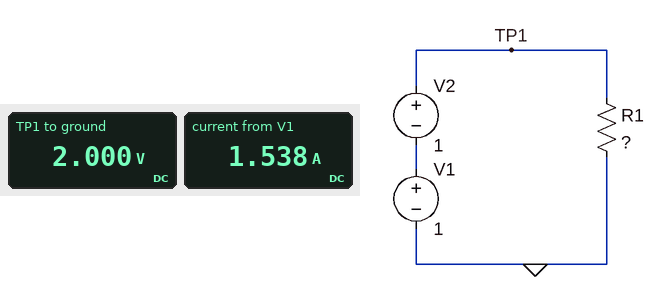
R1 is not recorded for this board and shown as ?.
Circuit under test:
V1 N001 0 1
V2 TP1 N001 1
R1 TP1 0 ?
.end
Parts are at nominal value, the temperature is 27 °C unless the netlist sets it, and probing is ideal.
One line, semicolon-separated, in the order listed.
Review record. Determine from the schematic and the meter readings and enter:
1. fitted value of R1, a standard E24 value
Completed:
1.3 Ω
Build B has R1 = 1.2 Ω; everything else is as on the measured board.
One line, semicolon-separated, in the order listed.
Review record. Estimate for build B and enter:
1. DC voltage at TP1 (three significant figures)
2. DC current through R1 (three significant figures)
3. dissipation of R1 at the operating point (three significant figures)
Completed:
2.00 V; 1.67 A; 3.33 W
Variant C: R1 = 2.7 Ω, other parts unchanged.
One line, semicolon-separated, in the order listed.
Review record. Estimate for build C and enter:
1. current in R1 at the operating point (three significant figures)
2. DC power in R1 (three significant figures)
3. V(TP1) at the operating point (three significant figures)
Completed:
741 mA; 1.48 W; 2.00 V
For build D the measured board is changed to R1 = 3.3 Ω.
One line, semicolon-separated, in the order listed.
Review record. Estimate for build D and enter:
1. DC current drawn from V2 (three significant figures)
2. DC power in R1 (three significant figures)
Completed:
606 mA; 1.21 W
